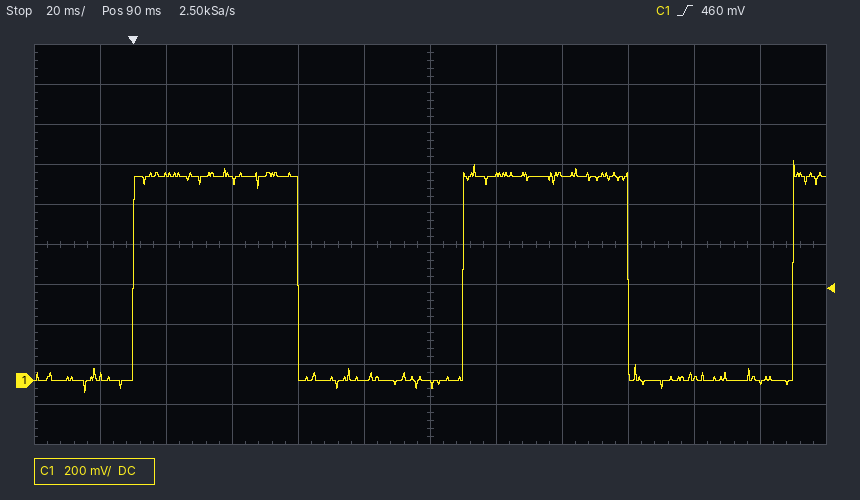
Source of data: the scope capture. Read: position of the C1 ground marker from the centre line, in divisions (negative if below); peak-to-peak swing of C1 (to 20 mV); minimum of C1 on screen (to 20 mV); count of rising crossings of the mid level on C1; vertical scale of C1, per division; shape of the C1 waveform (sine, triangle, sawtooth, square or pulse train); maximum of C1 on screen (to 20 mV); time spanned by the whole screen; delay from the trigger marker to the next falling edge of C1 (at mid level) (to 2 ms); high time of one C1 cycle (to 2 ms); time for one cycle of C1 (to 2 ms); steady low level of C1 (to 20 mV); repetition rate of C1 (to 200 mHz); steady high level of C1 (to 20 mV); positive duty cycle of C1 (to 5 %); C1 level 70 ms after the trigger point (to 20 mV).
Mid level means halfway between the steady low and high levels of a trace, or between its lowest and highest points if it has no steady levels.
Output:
-3.4 div
1.16 V
-60 mV
3
200 mV
square
1.10 V
240 ms
50 ms
50 ms
100 ms
0 mV
10.0 Hz
1.02 V
50 %
0 mV
